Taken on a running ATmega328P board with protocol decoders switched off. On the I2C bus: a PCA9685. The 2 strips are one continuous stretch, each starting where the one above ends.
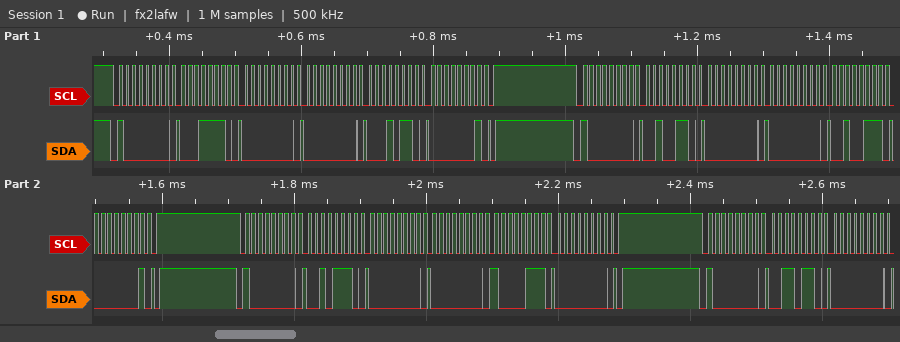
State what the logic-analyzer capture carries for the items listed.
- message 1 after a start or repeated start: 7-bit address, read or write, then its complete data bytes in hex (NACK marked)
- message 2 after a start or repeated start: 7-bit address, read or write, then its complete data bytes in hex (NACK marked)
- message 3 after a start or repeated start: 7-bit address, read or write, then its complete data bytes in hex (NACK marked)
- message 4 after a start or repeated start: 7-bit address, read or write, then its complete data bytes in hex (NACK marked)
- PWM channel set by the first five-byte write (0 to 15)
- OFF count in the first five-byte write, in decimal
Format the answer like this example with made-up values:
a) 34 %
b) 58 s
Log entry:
a) 0x40 write: 1E 00 00 16 01
b) 0x40 write: 26 00 00 27 01
c) 0x40 write: 2E 00 00 87 00
d) 0x40 write: 36 00
e) 6
f) 278
